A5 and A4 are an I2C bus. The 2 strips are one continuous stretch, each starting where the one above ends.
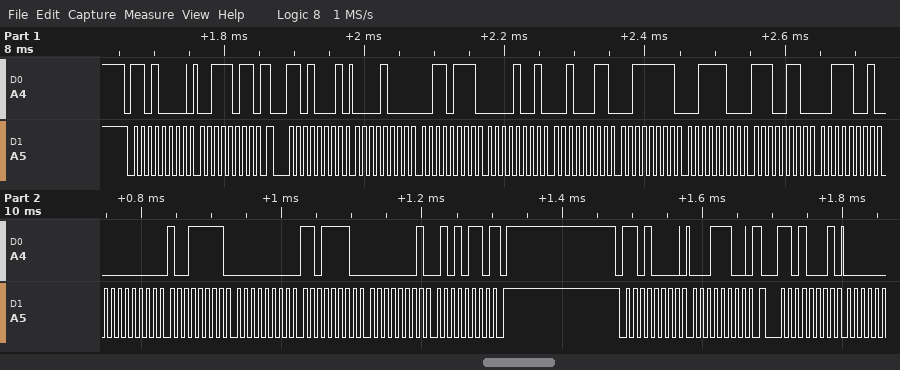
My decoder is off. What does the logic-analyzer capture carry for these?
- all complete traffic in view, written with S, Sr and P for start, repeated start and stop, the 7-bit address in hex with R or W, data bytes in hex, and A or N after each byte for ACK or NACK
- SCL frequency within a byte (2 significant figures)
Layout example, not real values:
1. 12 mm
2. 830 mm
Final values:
1. S 68W A 3B A Sr 68R A 08 A 37 A 09 A 23 A 3F A 3C A E6 A 39 A 00 A 9F A 00 A DE A 01 A 56 N P S 68W A 1C A Sr 68R A
2. 100 kHz
